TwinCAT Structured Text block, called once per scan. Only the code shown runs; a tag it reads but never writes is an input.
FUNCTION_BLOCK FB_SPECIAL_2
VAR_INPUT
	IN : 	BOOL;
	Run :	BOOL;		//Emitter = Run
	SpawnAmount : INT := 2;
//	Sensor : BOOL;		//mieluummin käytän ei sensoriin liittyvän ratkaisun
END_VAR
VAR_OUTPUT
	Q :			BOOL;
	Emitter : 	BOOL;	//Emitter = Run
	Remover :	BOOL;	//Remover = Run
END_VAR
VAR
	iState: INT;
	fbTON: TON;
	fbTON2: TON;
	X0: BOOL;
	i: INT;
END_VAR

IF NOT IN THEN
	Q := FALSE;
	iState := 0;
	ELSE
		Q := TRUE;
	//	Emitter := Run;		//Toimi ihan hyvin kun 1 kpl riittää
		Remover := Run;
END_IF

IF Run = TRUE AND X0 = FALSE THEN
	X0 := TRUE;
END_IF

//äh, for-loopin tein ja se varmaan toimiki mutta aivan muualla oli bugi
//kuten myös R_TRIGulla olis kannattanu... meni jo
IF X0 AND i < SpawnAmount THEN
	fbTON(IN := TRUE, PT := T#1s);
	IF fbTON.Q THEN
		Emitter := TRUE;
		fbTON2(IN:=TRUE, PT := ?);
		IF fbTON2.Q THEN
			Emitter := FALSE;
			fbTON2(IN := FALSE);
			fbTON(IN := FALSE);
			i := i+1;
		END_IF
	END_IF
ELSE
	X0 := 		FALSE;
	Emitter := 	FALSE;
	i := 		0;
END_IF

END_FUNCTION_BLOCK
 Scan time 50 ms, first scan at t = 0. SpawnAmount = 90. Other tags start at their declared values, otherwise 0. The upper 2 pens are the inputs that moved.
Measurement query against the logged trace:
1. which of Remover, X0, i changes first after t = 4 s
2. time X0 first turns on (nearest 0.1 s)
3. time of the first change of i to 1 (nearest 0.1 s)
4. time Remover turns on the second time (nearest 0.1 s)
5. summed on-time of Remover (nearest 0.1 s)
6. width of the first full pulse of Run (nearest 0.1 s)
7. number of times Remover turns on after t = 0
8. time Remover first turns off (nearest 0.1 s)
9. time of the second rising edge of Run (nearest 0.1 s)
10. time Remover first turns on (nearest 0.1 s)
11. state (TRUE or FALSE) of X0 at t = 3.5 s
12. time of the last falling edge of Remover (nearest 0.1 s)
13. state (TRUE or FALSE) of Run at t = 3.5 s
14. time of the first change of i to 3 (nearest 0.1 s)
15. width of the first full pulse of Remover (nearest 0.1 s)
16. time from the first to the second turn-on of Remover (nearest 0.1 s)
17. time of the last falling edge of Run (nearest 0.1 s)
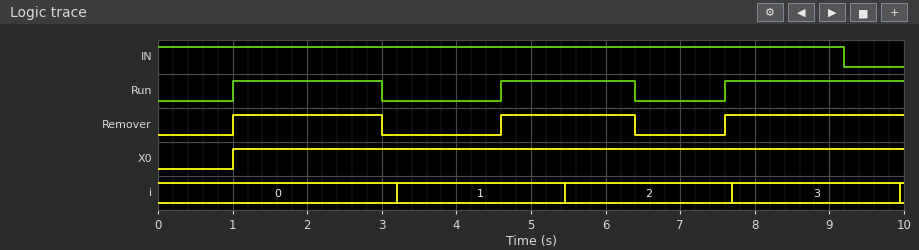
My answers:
Remover
1.0 s
3.2 s
4.6 s
6.2 s
2.0 s
3
3.0 s
4.6 s
1.0 s
TRUE
6.4 s
FALSE
7.7 s
2.0 s
3.6 s
6.4 s
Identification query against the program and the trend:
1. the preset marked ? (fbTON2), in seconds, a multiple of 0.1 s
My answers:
1.2 s
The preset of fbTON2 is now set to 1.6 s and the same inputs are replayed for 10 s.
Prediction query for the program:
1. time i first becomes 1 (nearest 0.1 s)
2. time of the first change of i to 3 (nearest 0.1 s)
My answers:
3.6 s
8.9 s
